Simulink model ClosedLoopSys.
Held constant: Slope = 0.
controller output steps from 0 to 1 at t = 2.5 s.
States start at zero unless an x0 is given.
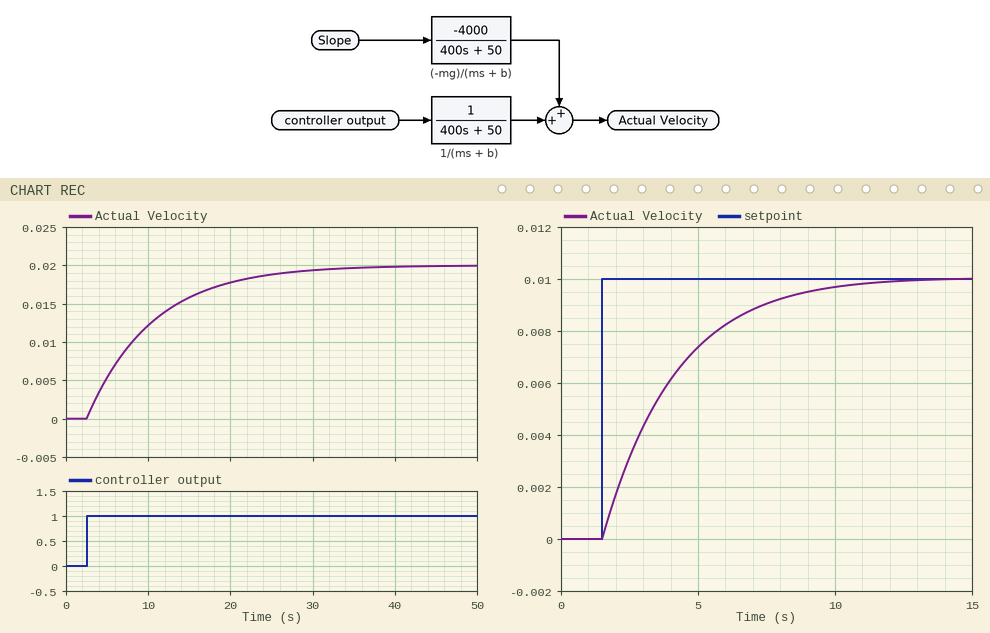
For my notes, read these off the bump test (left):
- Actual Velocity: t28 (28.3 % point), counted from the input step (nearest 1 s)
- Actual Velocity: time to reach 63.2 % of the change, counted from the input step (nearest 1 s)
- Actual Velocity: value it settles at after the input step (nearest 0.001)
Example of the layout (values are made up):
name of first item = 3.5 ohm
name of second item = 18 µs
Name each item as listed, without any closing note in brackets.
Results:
Actual Velocity: t28 (28.3 % point), counted from the input step = 3 s
Actual Velocity: time to reach 63.2 % of the change, counted from the input step = 8 s
Actual Velocity: value it settles at after the input step = 0.020
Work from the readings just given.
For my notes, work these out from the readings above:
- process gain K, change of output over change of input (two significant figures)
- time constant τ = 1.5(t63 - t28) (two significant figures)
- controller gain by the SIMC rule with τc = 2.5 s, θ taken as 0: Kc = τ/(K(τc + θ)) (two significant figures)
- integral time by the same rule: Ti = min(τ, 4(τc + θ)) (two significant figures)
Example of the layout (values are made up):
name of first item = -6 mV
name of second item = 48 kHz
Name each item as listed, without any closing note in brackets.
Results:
process gain K, change of output over change of input = 0.020
time constant τ = 1.5(t63 - t28) = 7.5 s
controller gain by the SIMC rule with τc = 2.5 s, θ taken as 0: Kc = τ/(K(τc + θ)) = 150
integral time by the same rule: Ti = min(τ, 4(τc + θ)) = 7.5 s
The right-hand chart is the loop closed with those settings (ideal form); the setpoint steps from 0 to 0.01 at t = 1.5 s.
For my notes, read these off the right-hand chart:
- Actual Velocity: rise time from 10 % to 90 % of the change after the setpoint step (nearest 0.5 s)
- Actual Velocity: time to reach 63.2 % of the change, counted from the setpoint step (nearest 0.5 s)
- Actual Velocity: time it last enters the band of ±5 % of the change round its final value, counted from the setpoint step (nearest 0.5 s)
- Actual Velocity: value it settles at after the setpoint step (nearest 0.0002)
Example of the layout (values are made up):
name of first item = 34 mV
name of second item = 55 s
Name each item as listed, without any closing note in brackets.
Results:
Actual Velocity: rise time from 10 % to 90 % of the change after the setpoint step = 5.5 s
Actual Velocity: time to reach 63.2 % of the change, counted from the setpoint step = 2.5 s
Actual Velocity: time it last enters the band of ±5 % of the change round its final value, counted from the setpoint step = 7.5 s
Actual Velocity: value it settles at after the setpoint step = 0.0100
